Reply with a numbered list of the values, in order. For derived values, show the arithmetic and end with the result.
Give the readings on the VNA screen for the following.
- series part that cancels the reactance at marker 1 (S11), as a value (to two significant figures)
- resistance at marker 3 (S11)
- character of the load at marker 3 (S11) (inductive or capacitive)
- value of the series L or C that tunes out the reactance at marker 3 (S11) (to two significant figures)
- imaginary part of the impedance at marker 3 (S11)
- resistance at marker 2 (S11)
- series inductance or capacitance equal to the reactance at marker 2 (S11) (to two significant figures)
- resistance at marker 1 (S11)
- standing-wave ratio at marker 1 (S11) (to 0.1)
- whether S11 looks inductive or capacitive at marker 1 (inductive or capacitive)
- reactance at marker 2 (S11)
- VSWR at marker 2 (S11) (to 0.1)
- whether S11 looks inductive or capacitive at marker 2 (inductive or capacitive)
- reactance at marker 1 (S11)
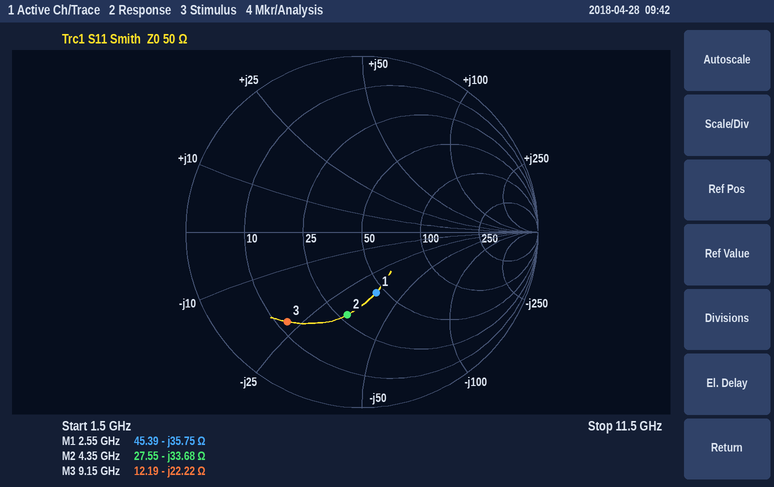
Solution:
1. L = 35.75 Ω/(2π × 2.55 GHz) ≈ 2.2 nH
2. 12.19 Ω
3. capacitive
4. L = 22.22 Ω/(2π × 9.15 GHz) ≈ 386 pH, so 390 pH to two significant figures
5. -22.22 Ω
6. 27.55 Ω
7. C = 1/(2π × 4.35 GHz × 33.68 Ω) ≈ 1.1 pF
8. 45.39 Ω
9. 2.1
10. capacitive
11. -33.68 Ω
12. 2.8
13. capacitive
14. -35.75 Ω
